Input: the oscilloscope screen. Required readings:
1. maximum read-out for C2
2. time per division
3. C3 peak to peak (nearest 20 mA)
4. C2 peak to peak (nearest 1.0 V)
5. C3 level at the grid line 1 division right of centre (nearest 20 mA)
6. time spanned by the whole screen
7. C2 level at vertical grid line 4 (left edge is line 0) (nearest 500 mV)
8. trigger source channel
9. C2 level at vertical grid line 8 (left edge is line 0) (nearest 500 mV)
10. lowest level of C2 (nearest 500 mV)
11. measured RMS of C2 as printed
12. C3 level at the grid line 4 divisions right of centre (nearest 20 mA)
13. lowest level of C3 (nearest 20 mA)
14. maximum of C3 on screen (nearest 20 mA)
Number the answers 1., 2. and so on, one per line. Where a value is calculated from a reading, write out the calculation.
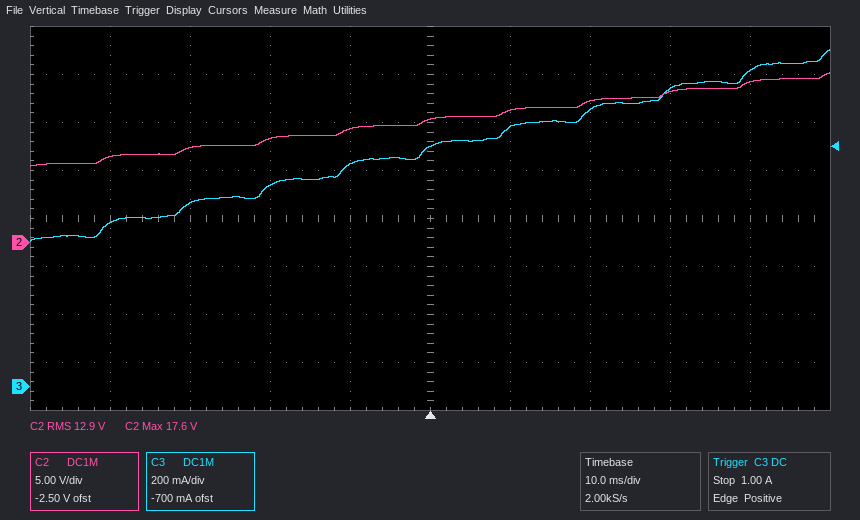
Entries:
1. 17.6 V
2. 10 ms
3. 1.40 A − (600 mA) = 800 mA
4. 10.0 V
5. 1.08 A
6. 100 ms
7. 12.0 V
8. C3
9. 15.5 V
10. 8.0 V
11. 12.9 V
12. 1.32 A
13. 600 mA
14. 1.40 A
